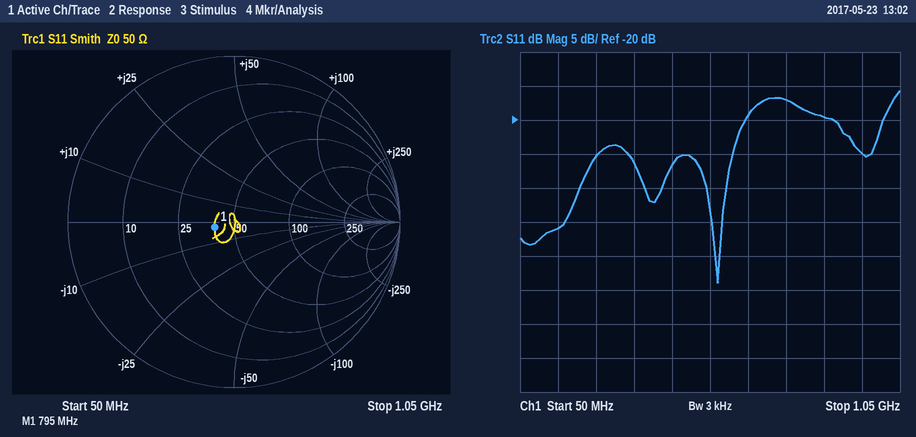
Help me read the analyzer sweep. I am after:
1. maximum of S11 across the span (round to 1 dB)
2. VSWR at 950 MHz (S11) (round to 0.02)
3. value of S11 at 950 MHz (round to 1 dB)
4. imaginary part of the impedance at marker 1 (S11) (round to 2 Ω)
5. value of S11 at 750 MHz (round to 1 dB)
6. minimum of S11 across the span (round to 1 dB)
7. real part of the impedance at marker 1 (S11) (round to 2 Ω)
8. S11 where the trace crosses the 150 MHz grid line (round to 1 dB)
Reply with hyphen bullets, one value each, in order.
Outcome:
- -16 dB
- 1.12
- -25 dB
- -2 Ω
- -17 dB
- -44 dB
- 40 Ω
- -36 dB
